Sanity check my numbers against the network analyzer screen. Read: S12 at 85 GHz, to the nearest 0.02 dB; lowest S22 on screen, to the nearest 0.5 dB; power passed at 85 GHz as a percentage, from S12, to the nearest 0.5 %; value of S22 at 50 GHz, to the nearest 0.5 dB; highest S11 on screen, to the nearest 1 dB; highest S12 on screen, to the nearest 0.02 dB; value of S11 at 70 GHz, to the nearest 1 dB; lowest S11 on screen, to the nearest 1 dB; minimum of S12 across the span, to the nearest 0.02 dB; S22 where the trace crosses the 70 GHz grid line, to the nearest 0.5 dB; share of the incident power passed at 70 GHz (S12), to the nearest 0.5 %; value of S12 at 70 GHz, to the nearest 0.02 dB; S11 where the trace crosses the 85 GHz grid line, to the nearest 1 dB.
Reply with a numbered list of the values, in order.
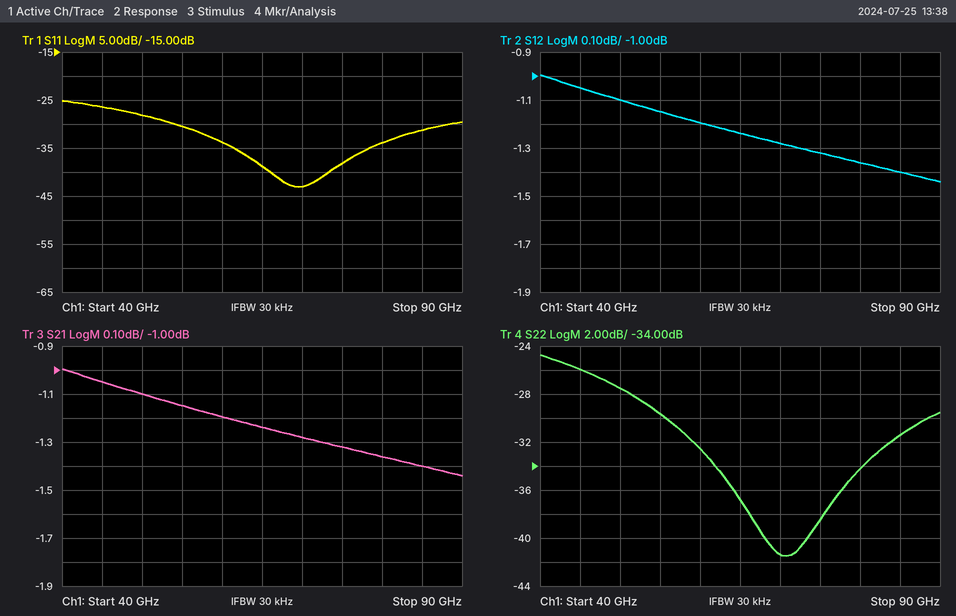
1. -1.40 dB
2. -41.5 dB
3. 72.5 %
4. -27.5 dB
5. -25 dB
6. -1.00 dB
7. -43 dB
8. -43 dB
9. -1.44 dB
10. -41.5 dB
11. 74.5 %
12. -1.28 dB
13. -31 dB
